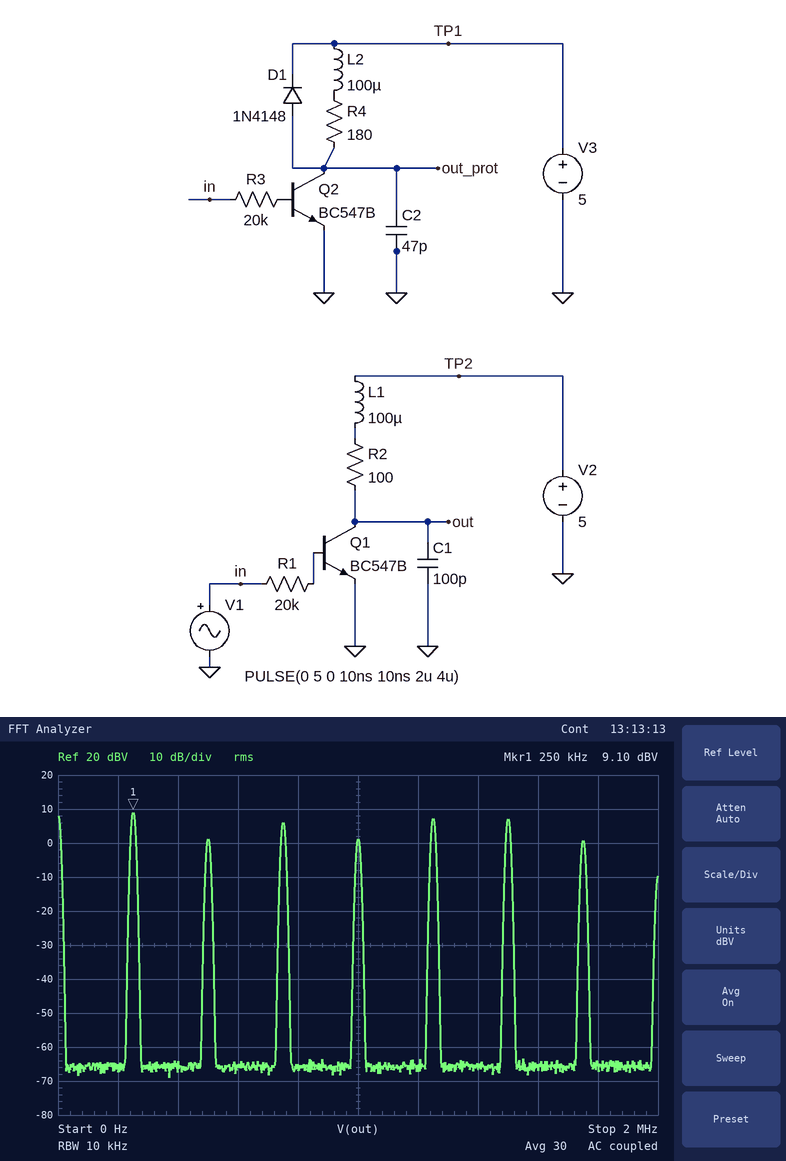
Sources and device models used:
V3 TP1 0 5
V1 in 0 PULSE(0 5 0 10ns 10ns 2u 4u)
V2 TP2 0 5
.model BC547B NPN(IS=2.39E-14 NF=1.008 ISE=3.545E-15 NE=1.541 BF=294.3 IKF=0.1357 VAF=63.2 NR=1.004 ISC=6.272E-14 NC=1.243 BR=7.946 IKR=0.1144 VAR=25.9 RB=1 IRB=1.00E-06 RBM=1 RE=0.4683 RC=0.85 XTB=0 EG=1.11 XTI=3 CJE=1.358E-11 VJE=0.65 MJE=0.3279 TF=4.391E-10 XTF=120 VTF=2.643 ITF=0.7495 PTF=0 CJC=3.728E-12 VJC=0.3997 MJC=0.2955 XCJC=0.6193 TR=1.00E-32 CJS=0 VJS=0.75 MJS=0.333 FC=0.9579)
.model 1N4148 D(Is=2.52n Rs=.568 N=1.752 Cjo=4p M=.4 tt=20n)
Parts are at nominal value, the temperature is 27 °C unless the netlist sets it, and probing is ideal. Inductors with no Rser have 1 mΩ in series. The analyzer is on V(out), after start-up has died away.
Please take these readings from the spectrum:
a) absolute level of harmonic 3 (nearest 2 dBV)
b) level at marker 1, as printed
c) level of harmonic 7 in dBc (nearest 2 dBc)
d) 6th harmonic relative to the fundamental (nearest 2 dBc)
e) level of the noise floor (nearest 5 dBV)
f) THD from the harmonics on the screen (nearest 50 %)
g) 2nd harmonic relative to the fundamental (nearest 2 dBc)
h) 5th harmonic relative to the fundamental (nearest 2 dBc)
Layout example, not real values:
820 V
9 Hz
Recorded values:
6 dBV
9.10 dBV
-8 dBc
-2 dBc
-65 dBV
150 %
-8 dBc
-2 dBc
